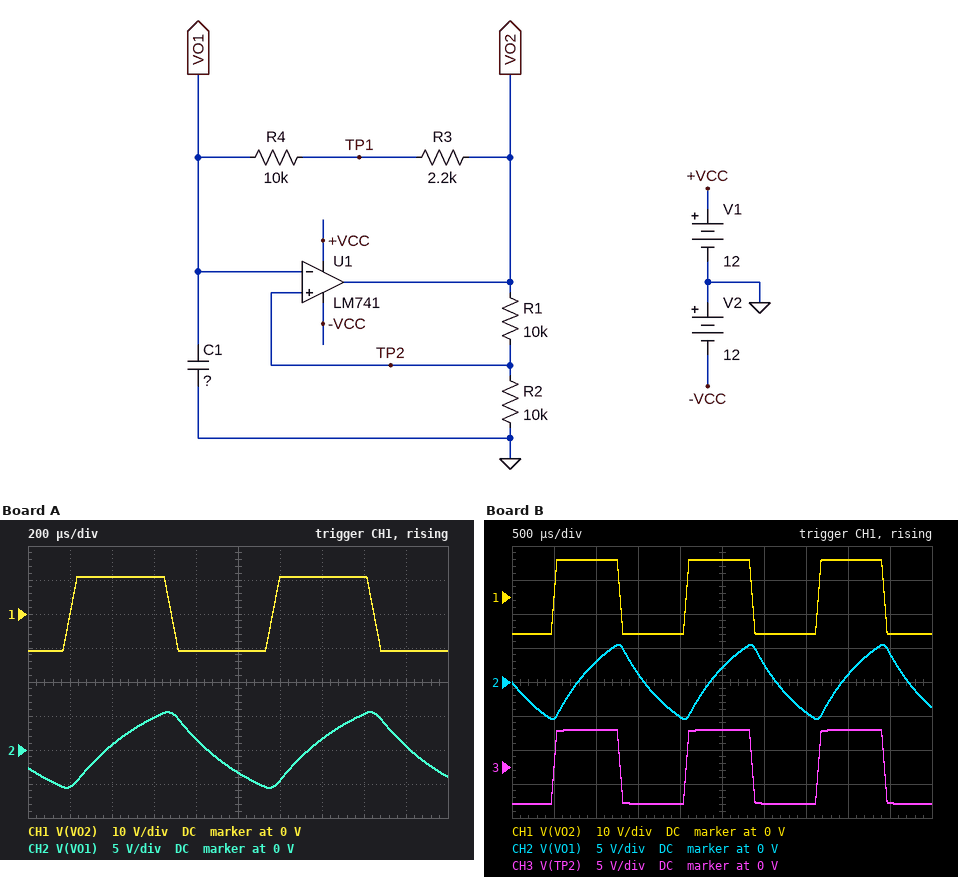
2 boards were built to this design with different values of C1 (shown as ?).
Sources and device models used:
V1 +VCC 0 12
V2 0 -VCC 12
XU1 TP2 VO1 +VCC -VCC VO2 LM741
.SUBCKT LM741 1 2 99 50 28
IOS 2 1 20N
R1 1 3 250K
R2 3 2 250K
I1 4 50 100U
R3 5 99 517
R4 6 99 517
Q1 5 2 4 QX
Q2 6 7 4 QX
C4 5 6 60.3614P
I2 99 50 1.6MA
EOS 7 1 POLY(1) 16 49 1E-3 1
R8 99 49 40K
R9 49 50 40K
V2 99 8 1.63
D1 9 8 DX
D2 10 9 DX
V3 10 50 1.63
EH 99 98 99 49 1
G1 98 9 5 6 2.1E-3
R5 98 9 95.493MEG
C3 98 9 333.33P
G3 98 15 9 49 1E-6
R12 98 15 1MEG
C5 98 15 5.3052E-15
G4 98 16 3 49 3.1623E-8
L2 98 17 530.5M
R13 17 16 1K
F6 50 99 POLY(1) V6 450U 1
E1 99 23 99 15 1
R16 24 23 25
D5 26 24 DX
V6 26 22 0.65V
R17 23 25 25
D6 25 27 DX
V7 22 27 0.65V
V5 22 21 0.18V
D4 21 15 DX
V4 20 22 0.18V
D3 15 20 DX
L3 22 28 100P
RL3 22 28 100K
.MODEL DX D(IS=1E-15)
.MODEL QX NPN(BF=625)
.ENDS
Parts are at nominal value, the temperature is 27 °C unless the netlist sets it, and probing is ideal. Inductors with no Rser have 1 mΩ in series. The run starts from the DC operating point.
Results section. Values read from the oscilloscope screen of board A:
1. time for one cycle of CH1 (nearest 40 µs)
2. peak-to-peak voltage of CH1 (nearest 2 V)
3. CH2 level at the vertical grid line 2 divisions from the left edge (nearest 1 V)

960 µs
22 V
1 V
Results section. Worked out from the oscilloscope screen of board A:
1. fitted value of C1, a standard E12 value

33 nF
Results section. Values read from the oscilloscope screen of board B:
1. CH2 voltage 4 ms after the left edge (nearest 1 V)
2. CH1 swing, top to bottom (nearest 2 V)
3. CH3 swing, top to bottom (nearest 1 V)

1 V
22 V
11 V
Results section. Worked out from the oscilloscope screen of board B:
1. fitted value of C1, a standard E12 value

56 nF
